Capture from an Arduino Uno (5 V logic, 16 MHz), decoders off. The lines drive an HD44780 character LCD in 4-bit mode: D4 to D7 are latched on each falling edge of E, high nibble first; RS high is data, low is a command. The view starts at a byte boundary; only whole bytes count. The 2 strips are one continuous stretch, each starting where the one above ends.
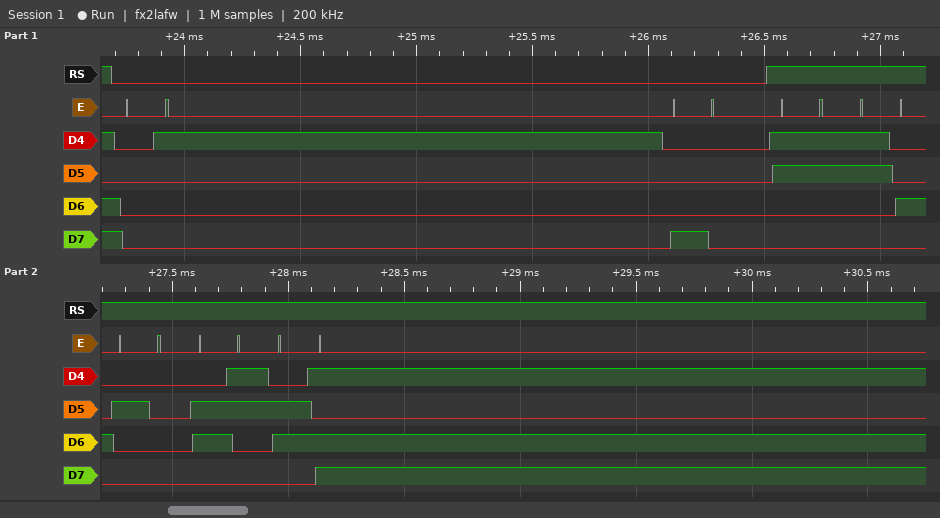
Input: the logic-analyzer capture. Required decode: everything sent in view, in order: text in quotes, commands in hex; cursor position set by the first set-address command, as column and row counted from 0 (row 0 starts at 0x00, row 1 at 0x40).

0x01 0x80 "34 cm"
column 0, row 0
